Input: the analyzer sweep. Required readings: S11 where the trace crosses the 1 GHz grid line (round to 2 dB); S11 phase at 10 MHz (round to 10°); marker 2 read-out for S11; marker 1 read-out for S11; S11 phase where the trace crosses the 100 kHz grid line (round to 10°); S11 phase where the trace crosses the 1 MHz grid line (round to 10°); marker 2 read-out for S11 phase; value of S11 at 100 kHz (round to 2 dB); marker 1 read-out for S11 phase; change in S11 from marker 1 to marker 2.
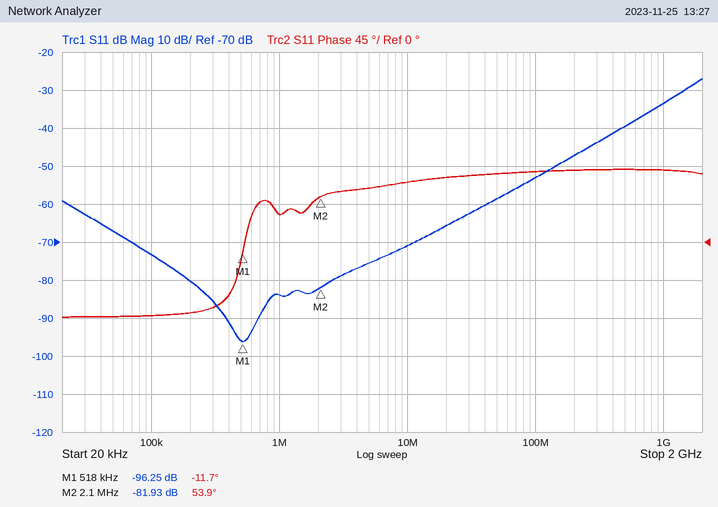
-34 dB
70°
-81.93 dB
-96.25 dB
-90°
30°
53.9°
-74 dB
-11.7°
14.32 dB
